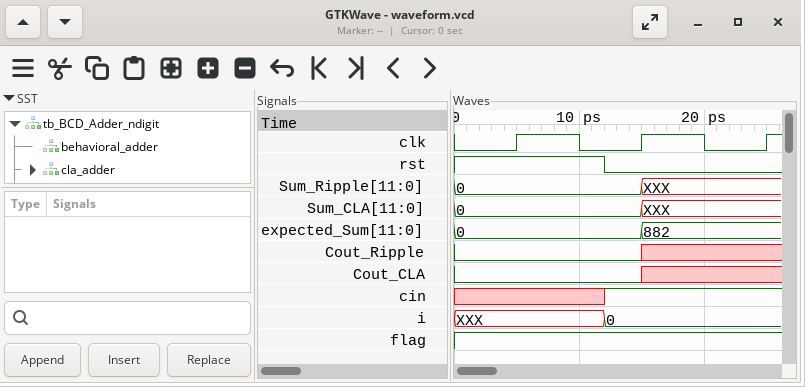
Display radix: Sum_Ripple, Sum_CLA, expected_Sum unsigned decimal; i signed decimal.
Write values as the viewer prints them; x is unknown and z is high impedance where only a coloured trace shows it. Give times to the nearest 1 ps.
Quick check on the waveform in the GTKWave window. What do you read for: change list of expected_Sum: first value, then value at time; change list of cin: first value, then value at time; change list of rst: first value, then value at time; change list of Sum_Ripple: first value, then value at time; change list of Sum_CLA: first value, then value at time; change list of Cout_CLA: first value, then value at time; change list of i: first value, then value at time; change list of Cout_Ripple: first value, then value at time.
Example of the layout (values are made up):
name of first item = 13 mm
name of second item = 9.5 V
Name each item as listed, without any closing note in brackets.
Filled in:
change list of expected_Sum: first value, then value at time = 0, 882 at 15 ps
change list of cin: first value, then value at time = x, 1 at 12 ps
change list of rst: first value, then value at time = 1, 0 at 12 ps
change list of Sum_Ripple: first value, then value at time = 0, XXX at 15 ps
change list of Sum_CLA: first value, then value at time = 0, XXX at 15 ps
change list of Cout_CLA: first value, then value at time = 0, x at 15 ps
change list of i: first value, then value at time = XXX, 0 at 12 ps
change list of Cout_Ripple: first value, then value at time = 0, x at 15 ps
